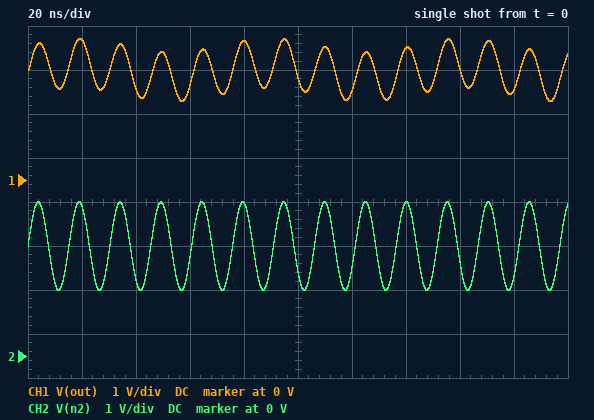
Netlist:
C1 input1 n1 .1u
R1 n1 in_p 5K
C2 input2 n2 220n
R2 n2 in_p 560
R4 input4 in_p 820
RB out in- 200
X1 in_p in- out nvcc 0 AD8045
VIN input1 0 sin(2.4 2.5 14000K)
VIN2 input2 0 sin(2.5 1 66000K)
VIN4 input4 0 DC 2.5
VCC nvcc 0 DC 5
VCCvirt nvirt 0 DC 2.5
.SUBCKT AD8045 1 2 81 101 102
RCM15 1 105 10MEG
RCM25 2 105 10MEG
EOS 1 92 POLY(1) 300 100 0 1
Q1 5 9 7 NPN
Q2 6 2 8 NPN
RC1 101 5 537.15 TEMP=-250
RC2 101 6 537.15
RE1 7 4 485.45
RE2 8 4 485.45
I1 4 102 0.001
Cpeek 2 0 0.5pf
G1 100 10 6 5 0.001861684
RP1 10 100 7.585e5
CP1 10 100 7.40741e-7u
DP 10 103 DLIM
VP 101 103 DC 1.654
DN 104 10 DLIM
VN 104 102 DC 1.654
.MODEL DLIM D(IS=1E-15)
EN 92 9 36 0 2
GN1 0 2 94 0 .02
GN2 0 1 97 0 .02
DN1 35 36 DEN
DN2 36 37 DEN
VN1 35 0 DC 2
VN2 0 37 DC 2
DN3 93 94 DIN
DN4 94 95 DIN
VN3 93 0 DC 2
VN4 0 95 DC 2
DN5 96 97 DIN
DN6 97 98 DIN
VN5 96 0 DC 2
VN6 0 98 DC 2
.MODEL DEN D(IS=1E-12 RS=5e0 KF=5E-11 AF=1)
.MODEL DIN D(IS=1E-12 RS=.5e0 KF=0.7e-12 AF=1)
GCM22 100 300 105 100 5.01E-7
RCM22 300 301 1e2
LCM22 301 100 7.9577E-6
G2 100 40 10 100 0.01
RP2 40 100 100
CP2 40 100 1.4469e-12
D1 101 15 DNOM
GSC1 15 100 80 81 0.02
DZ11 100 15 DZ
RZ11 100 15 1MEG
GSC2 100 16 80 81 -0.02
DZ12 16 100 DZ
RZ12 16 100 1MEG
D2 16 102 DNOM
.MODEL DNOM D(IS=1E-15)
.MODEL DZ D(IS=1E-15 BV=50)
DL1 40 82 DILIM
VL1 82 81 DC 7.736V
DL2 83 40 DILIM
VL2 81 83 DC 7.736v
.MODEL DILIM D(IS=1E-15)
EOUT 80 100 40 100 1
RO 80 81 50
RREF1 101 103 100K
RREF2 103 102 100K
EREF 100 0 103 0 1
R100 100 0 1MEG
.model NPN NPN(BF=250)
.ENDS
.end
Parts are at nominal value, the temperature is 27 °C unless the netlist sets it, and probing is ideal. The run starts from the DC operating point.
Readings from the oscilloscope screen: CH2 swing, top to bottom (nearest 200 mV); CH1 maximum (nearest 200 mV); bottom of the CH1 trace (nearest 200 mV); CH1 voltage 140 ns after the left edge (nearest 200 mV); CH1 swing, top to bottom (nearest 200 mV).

2.0 V
3.2 V
1.8 V
3.0 V
1.4 V
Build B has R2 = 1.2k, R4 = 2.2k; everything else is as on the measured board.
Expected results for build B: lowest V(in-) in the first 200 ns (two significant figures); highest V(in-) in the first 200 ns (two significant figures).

1.6 V
3.4 V
